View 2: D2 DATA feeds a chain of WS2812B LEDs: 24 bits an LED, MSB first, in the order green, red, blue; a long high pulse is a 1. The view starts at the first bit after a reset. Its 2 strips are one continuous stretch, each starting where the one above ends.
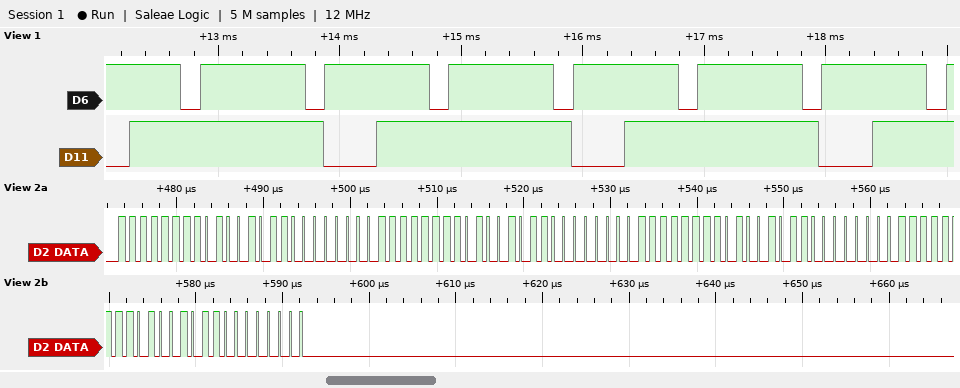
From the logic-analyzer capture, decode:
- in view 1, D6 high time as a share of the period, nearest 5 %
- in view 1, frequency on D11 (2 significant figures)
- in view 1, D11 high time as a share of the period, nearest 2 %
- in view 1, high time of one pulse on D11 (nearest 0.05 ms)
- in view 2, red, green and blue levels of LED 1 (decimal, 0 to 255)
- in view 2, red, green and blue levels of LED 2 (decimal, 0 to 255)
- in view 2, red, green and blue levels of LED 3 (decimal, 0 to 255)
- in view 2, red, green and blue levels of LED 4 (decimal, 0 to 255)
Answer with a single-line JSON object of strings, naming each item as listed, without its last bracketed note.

{"in view 1, D6 high time as a share of the period, nearest 5 %": "85 %", "in view 1, frequency on D11": "490 Hz", "in view 1, D11 high time as a share of the period, nearest 2 %": "78 %", "in view 1, high time of one pulse on D11": "1.60 ms", "in view 2, red, green and blue levels of LED 1": "75, 255, 0", "in view 2, red, green and blue levels of LED 2": "75, 255, 0", "in view 2, red, green and blue levels of LED 3": "75, 255, 0", "in view 2, red, green and blue levels of LED 4": "75, 255, 0"}
